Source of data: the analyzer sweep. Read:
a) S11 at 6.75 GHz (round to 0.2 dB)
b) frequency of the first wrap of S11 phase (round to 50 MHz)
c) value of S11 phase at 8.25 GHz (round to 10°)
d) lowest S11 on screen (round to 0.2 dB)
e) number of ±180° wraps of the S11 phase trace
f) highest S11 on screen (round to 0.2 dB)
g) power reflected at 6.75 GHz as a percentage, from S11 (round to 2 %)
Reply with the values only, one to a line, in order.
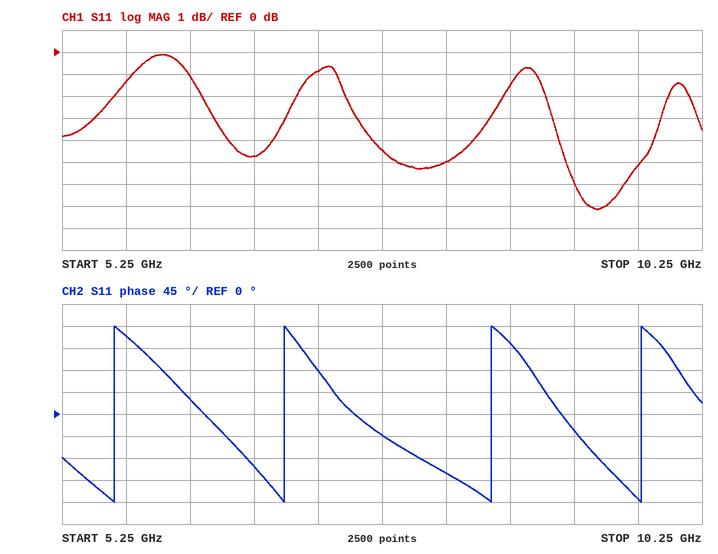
-4.8 dB
5.65 GHz
-120°
-7.2 dB
4
-0.2 dB
34 %
